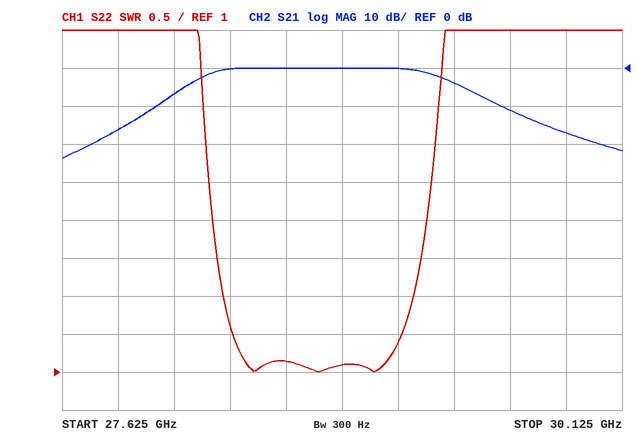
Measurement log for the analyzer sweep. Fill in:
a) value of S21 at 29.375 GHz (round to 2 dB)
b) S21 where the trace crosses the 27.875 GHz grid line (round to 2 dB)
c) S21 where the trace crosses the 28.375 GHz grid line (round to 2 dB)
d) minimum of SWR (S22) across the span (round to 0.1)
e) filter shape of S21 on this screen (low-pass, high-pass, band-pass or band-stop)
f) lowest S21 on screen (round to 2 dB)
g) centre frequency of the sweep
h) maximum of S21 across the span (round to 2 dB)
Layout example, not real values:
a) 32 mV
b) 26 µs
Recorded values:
a) -4 dB
b) -16 dB
c) 0 dB
d) 1.0
e) band-pass
f) -24 dB
g) 28.875 GHz
h) 0 dB
